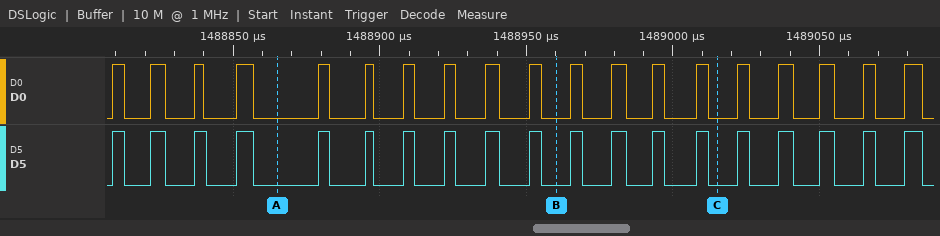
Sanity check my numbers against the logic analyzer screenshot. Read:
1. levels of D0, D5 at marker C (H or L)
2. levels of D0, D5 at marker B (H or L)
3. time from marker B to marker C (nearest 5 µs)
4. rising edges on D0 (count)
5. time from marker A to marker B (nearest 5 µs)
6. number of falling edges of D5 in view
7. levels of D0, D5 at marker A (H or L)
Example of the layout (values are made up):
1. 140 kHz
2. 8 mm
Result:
1. D0=L, D5=L
2. D0=L, D5=L
3. 55 µs
4. 19
5. 95 µs
6. 19
7. D0=L, D5=L
